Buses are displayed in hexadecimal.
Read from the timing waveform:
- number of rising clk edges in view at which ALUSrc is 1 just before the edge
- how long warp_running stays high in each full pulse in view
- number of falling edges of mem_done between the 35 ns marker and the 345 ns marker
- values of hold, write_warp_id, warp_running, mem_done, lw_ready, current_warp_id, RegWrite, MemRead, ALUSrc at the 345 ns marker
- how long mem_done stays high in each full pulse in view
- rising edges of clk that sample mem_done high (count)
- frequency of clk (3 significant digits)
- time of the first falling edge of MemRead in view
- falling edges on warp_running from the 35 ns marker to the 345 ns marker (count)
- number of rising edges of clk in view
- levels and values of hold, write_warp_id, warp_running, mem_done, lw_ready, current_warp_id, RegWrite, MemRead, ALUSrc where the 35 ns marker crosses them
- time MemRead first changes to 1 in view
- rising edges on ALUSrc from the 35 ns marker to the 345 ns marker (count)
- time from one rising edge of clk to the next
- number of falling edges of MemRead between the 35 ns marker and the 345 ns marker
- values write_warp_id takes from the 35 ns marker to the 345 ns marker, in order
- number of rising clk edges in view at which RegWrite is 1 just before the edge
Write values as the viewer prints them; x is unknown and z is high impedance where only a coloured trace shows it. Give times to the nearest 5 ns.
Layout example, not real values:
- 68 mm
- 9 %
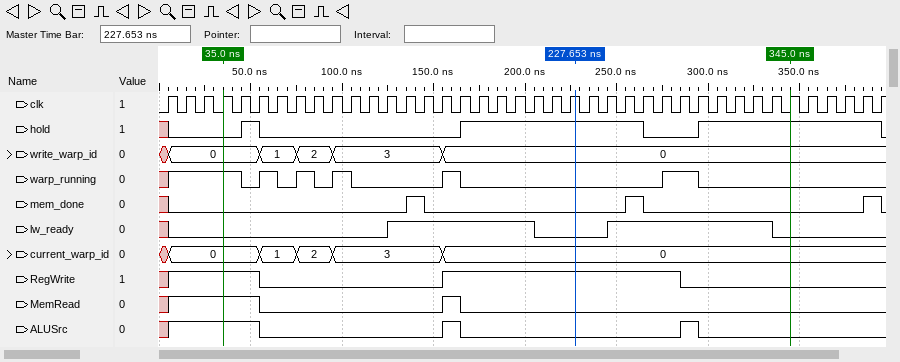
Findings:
- 7
- 10 ns, 10 ns, 10 ns, 10 ns, 20 ns
- 2
- hold=1, write_warp_id=0, warp_running=0, mem_done=0, lw_ready=0, current_warp_id=0, RegWrite=0, MemRead=0, ALUSrc=0
- 10 ns, 10 ns, 10 ns
- 3
- 100 MHz
- 55 ns
- 6
- 40
- hold=0, write_warp_id=0, warp_running=1, mem_done=0, lw_ready=0, current_warp_id=0, RegWrite=1, MemRead=1, ALUSrc=1
- 5 ns
- 2
- 10 ns
- 2
- 0, 1, 2, 3, 0
- 18
